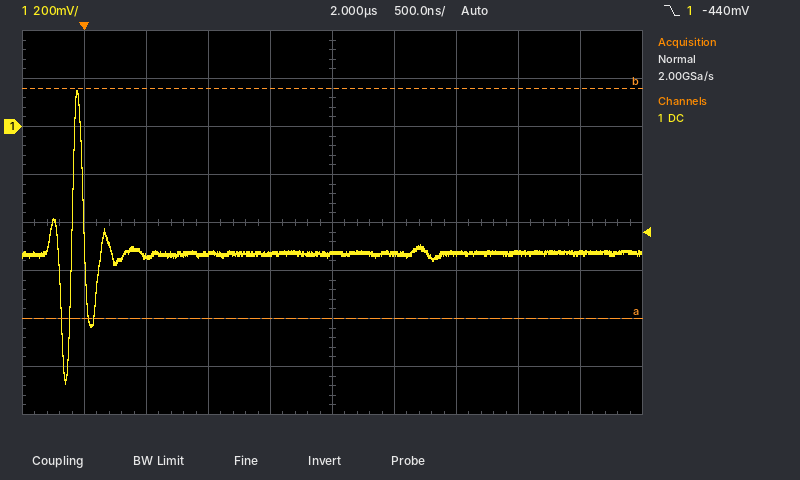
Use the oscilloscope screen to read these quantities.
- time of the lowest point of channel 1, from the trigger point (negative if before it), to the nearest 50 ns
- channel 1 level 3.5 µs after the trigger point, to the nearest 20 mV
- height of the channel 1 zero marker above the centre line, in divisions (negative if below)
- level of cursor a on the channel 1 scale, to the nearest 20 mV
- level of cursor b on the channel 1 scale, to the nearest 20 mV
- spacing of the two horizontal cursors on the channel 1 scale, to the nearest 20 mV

-150 ns
-520 mV
+2.0 div
-800 mV
160 mV
960 mV
